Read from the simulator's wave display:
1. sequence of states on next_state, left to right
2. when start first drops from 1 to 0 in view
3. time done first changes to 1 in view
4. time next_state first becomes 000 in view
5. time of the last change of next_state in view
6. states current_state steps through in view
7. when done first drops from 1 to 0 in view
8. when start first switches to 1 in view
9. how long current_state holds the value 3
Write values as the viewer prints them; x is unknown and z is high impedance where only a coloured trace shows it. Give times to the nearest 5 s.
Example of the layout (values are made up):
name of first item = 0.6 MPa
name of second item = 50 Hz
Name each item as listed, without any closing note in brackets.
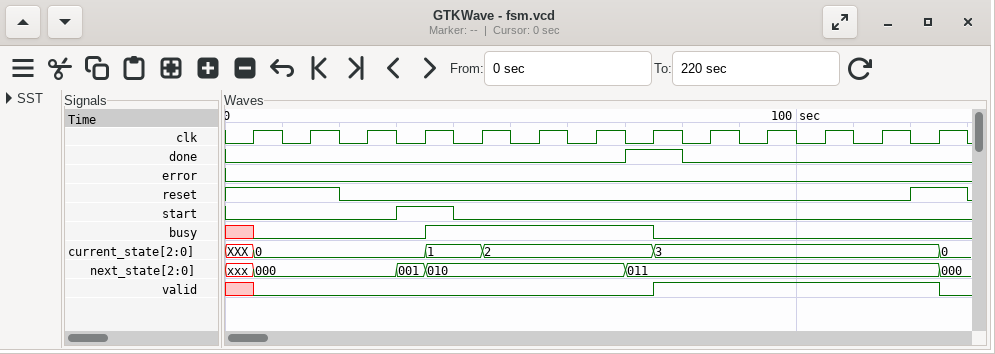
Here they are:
sequence of states on next_state, left to right = xxx, 000, 001, 010, 011, 000
when start first drops from 1 to 0 in view = 40 s
time done first changes to 1 in view = 70 s
time next_state first becomes 000 in view = 5 s
time of the last change of next_state in view = 125 s
states current_state steps through in view = XXX, 0, 1, 2, 3, 0
when done first drops from 1 to 0 in view = 80 s
when start first switches to 1 in view = 30 s
how long current_state holds the value 3 = 50 s
